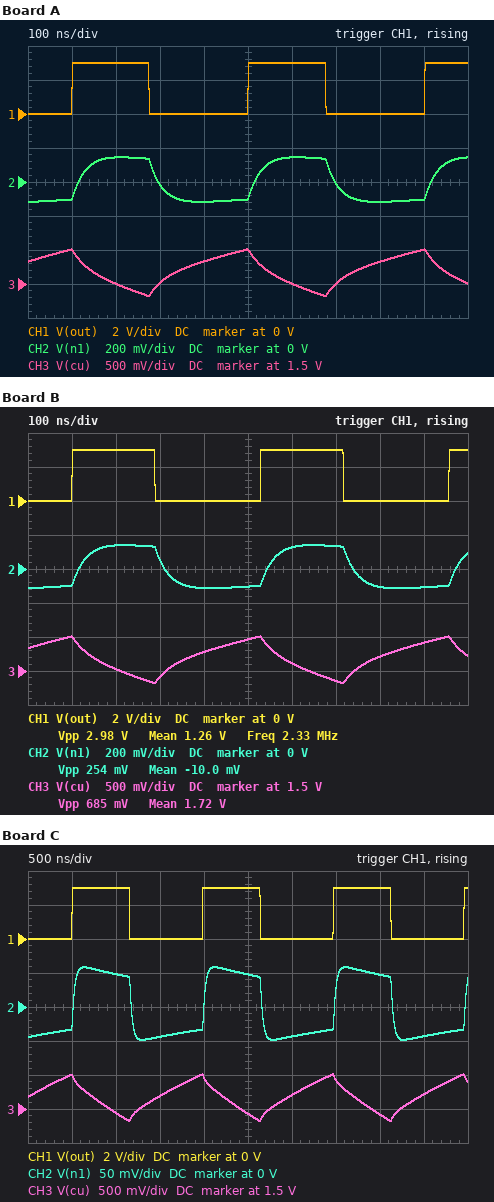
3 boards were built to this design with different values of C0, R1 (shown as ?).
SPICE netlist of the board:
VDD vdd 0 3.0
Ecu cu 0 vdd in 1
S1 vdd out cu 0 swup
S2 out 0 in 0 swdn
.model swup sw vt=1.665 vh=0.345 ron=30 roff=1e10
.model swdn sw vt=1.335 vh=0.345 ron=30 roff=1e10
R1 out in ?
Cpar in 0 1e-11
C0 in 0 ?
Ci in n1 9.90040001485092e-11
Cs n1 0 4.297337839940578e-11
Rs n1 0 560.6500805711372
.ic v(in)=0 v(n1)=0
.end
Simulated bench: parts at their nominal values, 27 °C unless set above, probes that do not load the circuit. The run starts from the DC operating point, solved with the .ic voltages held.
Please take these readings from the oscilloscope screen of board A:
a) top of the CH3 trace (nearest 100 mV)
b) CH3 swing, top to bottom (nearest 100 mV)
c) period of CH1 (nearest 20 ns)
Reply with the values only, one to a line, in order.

2.0 V
700 mV
400 ns
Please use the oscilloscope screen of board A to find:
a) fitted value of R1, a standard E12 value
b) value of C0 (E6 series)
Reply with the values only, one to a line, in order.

4.7 kΩ
10 pF
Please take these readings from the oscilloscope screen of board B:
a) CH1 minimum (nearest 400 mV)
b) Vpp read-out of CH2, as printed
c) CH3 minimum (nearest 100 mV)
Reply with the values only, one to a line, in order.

0 V
254 mV
1.3 V
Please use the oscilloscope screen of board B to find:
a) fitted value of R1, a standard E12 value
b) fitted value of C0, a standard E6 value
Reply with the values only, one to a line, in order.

4.7 kΩ
15 pF
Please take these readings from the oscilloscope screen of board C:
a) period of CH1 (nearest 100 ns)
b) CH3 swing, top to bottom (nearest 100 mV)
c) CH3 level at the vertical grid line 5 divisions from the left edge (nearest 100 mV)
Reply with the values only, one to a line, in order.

1.5 µs
700 mV
1.4 V
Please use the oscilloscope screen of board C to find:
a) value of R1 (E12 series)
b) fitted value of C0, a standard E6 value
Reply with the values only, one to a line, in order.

15 kΩ
3.3 pF
